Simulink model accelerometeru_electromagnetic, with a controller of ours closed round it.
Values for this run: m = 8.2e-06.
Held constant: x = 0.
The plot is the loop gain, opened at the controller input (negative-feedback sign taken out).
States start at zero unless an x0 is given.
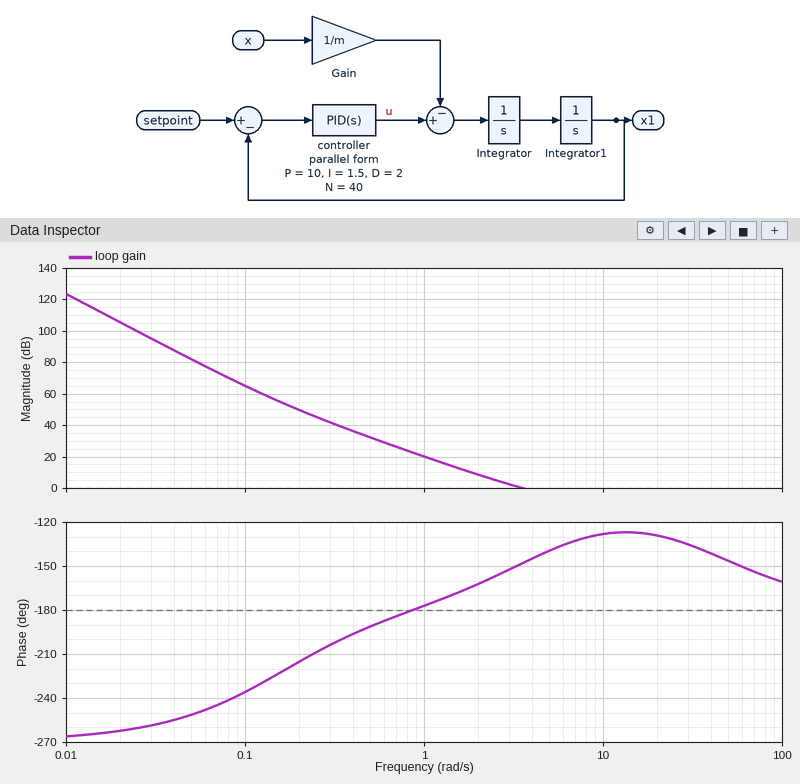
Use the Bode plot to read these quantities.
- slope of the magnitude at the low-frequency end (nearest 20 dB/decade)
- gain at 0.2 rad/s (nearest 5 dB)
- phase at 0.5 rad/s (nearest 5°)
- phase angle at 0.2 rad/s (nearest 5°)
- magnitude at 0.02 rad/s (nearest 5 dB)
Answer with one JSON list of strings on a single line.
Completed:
["-60 dB/decade", "50 dB", "-190°", "-215°", "105 dB"]
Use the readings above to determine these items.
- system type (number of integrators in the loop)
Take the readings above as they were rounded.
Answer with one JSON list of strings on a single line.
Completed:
["3"]
